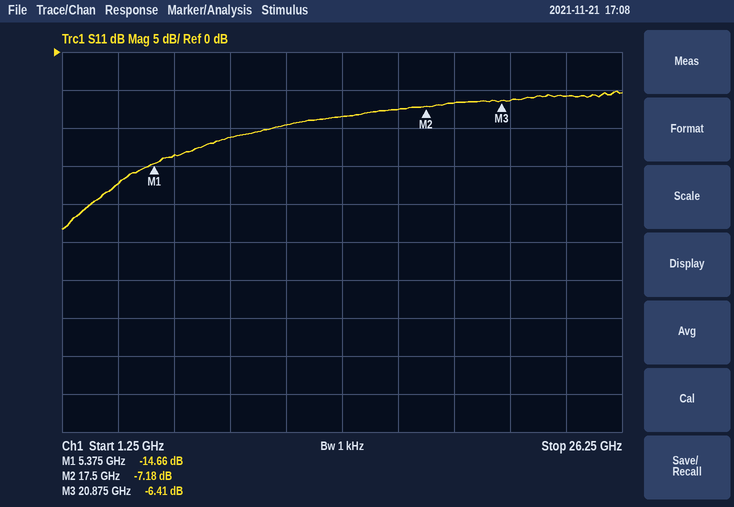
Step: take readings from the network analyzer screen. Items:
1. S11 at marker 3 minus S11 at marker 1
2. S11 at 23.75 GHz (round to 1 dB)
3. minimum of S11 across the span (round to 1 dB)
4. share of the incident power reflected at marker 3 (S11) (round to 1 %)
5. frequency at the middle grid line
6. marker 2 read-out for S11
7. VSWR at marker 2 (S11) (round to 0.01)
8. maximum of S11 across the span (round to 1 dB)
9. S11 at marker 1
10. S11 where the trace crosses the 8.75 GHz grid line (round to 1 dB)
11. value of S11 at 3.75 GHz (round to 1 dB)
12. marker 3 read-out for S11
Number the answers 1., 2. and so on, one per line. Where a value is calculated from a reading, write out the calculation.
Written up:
1. -6.41 − (-14.66) = 8.25 dB
2. -6 dB
3. -23 dB
4. 10^(-6.41/10) ≈ 23 %
5. 13.75 GHz
6. -7.18 dB
7. (1 + 0.4375)/(1 − 0.4375) ≈ 2.56
8. -5 dB
9. -14.66 dB
10. -11 dB
11. -17 dB
12. -6.41 dB
